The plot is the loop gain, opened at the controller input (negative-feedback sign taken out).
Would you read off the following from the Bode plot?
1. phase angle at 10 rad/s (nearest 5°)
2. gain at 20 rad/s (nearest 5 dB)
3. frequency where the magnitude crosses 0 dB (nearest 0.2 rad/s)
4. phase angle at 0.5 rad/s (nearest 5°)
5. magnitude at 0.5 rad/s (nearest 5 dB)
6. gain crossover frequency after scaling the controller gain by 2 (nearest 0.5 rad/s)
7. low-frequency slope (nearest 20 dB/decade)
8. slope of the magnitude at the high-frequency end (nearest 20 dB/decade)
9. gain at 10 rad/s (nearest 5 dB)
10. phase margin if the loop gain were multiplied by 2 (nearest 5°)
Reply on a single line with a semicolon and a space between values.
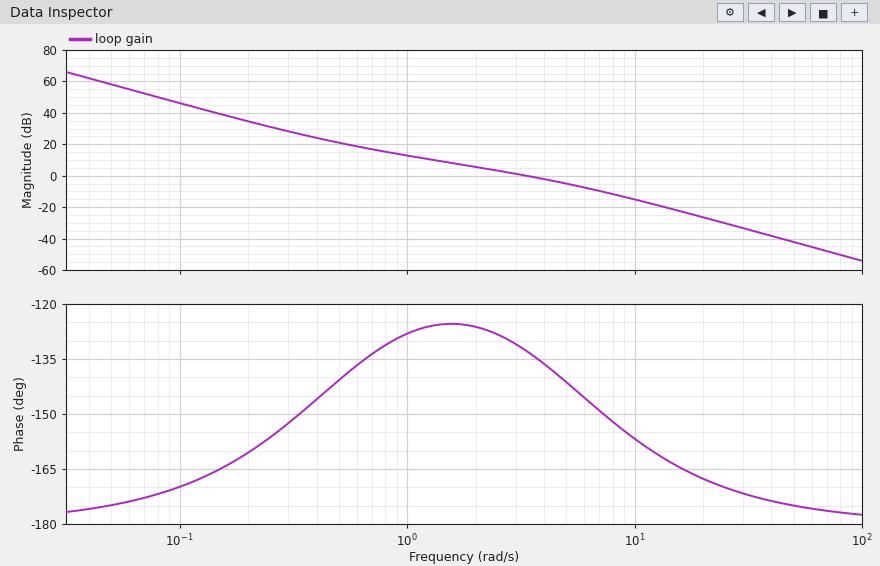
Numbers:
-155°; -25 dB; 3.4 rad/s; -140°; 20 dB; 5.5 rad/s; -40 dB/decade; -40 dB/decade; -15 dB; 35°
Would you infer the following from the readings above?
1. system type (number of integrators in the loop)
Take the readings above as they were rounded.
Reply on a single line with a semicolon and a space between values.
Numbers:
2
